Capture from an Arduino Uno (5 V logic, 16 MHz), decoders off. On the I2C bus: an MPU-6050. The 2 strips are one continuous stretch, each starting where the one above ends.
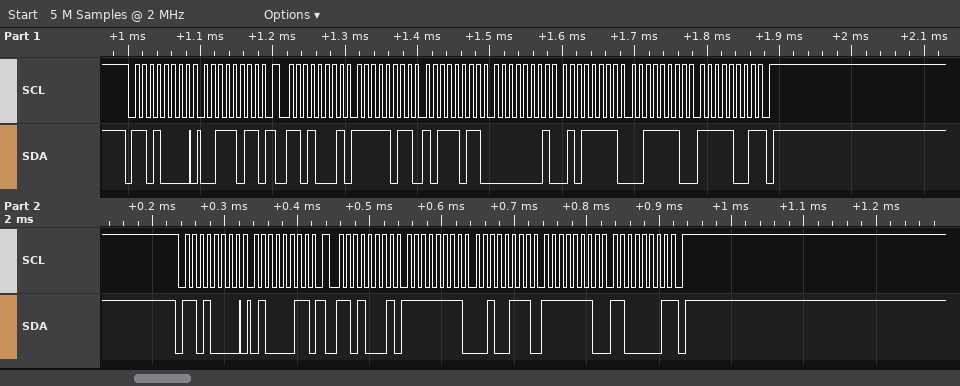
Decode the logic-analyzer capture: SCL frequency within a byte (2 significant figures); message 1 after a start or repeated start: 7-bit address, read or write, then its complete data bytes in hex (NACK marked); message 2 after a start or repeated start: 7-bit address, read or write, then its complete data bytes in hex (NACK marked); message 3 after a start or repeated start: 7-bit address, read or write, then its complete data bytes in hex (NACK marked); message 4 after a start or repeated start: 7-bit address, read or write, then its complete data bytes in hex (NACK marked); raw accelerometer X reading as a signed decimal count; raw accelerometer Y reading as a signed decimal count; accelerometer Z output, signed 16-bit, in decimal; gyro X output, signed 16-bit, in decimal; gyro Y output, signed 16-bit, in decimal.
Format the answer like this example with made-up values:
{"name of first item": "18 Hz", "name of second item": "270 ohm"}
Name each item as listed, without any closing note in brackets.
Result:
{"SCL frequency within a byte": "100 kHz", "message 1 after a start or repeated start: 7-bit address, read or write, then its complete data bytes in hex": "0x68 write: 3B", "message 2 after a start or repeated start: 7-bit address, read or write, then its complete data bytes in hex": "0x68 read: FB BB 01 5F 3E F9 NACK", "message 3 after a start or repeated start: 7-bit address, read or write, then its complete data bytes in hex": "0x68 write: 43", "message 4 after a start or repeated start: 7-bit address, read or write, then its complete data bytes in hex": "0x68 read: FF 27 FE C1 NACK", "raw accelerometer X reading as a signed decimal count": "-1093", "raw accelerometer Y reading as a signed decimal count": "351", "accelerometer Z output, signed 16-bit, in decimal": "16121", "gyro X output, signed 16-bit, in decimal": "-217", "gyro Y output, signed 16-bit, in decimal": "-319"}
